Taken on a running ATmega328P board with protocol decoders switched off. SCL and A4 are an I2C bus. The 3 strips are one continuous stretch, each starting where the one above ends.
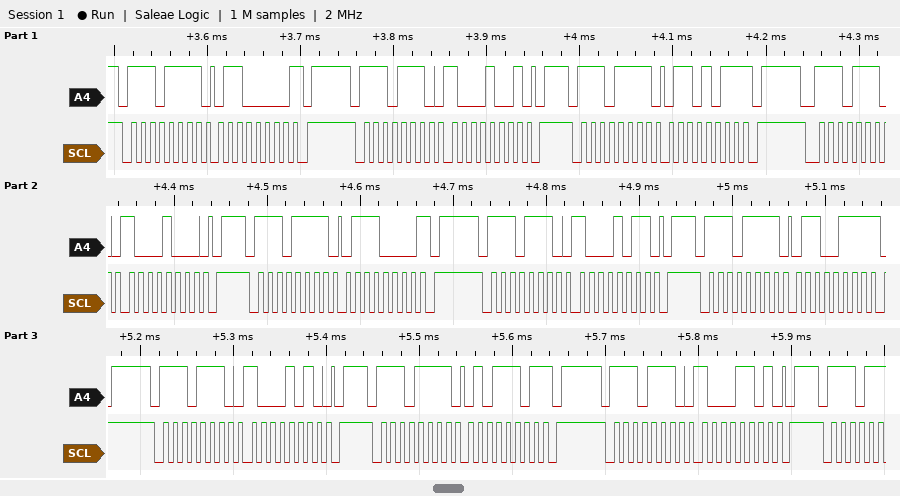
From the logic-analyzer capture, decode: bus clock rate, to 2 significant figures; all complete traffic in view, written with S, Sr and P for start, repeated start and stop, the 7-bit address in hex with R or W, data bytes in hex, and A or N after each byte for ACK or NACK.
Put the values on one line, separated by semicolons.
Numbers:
100 kHz; S 77R A 60 N P S 77W A 89 A P S 77R A 6B N P S 77W A 88 A P S 77R A 70 N P S 77W A 8B A P S 77R A 67 N P S 77W A 8A A P S 77R A 5D N P S 77W A 8D A P
